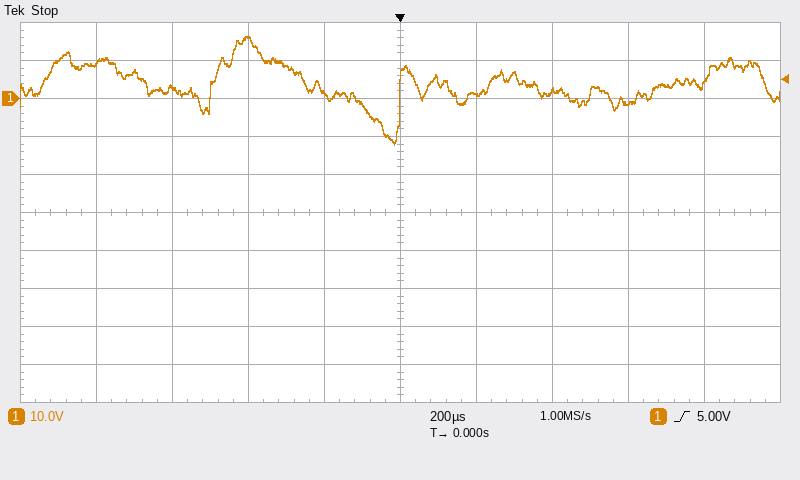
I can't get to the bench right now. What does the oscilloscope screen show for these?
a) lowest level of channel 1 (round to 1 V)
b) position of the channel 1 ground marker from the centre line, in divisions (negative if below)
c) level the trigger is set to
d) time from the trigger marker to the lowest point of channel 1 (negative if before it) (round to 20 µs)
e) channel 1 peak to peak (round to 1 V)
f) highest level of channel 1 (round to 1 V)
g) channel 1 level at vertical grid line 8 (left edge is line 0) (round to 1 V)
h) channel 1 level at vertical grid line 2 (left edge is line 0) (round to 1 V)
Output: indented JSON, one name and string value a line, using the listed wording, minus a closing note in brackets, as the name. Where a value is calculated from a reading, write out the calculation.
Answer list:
{
  "lowest level of channel 1": "-12 V",
  "position of the channel 1 ground marker from the centre line, in divisions": "+3.0 div",
  "level the trigger is set to": "5.00 V",
  "time from the trigger marker to the lowest point of channel 1 (negative if before it)": "-20 µs",
  "channel 1 peak to peak": "16 V − (-12 V) = 28 V",
  "highest level of channel 1": "16 V",
  "channel 1 level at vertical grid line 8 (left edge is line 0)": "-1 V",
  "channel 1 level at vertical grid line 2 (left edge is line 0)": "3 V"
}
